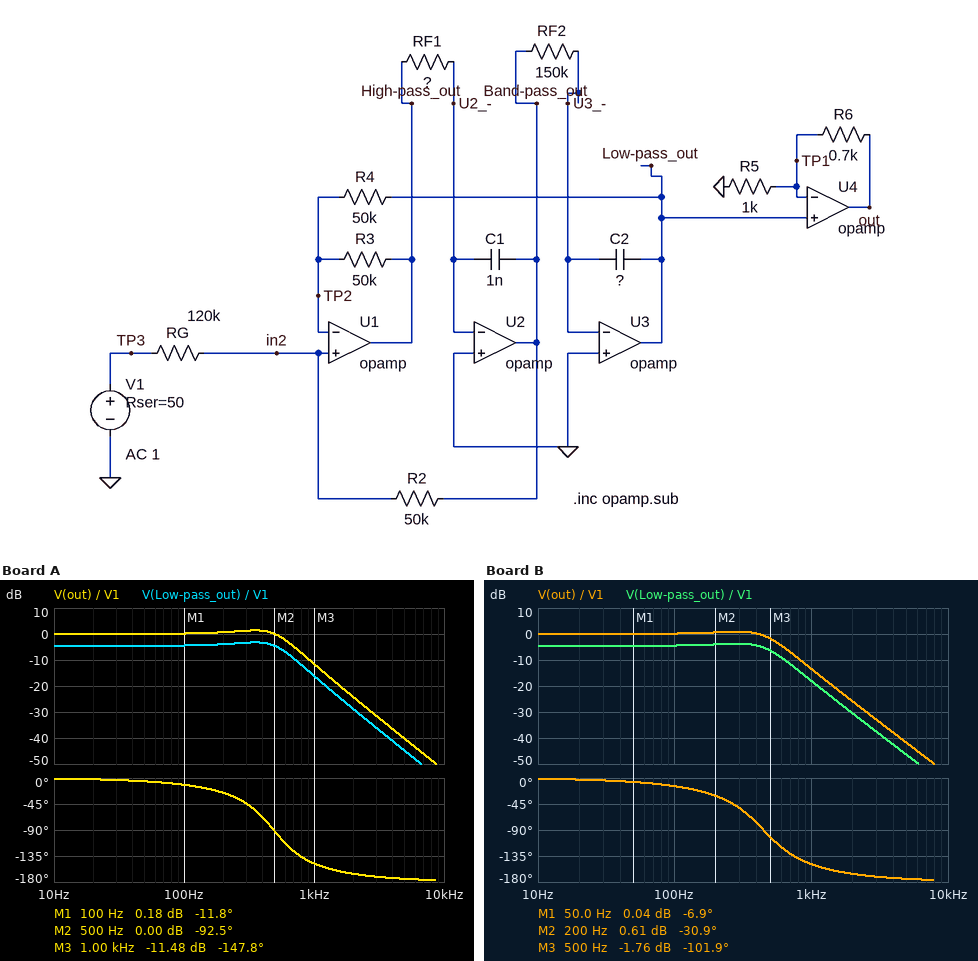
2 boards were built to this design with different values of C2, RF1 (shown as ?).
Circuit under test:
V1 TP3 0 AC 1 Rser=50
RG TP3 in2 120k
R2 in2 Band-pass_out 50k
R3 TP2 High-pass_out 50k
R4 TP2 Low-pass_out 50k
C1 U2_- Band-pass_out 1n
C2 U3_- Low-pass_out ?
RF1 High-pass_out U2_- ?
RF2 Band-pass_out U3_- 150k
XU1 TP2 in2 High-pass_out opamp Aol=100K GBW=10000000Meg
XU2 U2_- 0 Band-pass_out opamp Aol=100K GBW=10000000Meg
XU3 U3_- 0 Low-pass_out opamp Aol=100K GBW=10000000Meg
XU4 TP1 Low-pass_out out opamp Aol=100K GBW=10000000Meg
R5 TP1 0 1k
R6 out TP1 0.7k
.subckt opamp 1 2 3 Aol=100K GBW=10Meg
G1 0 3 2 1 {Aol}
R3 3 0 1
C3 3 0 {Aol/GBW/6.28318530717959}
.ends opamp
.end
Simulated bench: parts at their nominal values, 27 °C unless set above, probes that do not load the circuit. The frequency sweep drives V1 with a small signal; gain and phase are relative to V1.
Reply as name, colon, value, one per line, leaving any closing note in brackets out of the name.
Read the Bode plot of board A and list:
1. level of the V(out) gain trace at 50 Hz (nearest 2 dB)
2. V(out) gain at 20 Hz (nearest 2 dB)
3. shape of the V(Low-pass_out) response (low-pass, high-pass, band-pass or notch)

level of the V(out) gain trace at 50 Hz: 0 dB
V(out) gain at 20 Hz: 0 dB
shape of the V(Low-pass_out) response: low-pass
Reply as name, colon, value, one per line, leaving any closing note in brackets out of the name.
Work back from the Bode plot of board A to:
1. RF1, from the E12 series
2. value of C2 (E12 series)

RF1, from the E12 series: 470 kΩ
value of C2: 1.5 nF
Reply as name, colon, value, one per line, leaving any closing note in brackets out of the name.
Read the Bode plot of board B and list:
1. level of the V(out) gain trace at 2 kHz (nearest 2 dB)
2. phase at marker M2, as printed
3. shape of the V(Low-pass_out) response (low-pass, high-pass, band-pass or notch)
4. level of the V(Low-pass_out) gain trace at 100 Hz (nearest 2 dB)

level of the V(out) gain trace at 2 kHz: -26 dB
phase at marker M2, as printed: -30.9 deg
shape of the V(Low-pass_out) response: low-pass
level of the V(Low-pass_out) gain trace at 100 Hz: -4 dB
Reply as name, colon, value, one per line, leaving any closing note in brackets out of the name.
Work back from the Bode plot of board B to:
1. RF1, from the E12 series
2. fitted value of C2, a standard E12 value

RF1, from the E12 series: 470 kΩ
fitted value of C2, a standard E12 value: 1.8 nF
